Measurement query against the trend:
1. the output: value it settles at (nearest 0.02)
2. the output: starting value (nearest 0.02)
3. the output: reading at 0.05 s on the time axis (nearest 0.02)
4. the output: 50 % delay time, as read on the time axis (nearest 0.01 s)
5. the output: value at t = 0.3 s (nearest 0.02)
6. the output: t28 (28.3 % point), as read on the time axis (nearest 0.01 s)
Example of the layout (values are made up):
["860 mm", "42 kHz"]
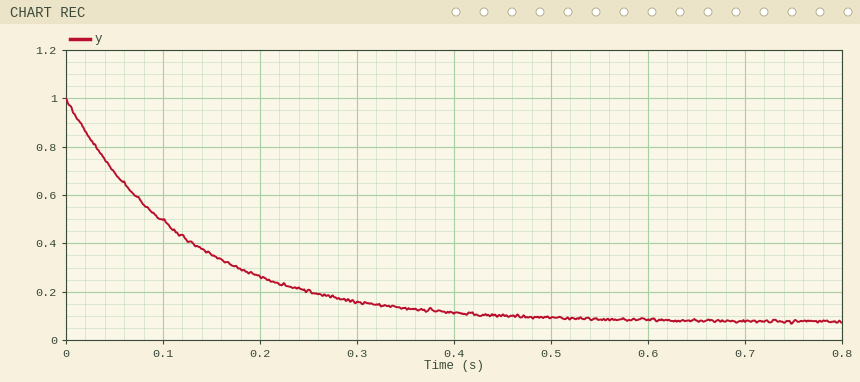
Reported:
["0.08", "1.00", "0.70", "0.09 s", "0.16", "0.04 s"]
